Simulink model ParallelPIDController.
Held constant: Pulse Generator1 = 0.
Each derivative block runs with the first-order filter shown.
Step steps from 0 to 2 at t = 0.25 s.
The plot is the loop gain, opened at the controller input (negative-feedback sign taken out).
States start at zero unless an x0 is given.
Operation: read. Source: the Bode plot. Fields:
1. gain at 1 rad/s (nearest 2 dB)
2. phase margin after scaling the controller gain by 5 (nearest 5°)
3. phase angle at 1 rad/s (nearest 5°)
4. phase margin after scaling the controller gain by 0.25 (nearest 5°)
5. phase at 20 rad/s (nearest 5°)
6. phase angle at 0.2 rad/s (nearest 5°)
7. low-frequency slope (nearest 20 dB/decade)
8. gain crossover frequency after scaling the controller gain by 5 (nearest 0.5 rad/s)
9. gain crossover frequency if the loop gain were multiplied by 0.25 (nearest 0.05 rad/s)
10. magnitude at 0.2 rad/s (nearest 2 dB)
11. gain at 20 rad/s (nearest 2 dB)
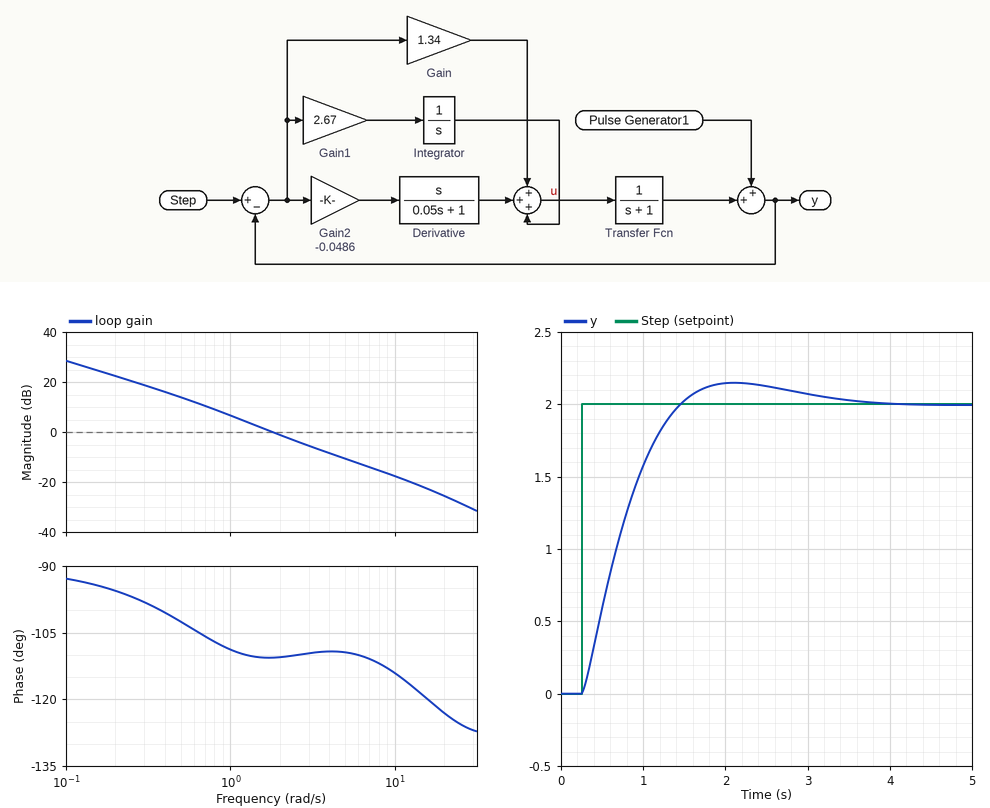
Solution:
6 dB
70°
-110°
75°
-125°
-95°
-20 dB/decade
7.0 rad/s
0.60 rad/s
22 dB
-26 dB
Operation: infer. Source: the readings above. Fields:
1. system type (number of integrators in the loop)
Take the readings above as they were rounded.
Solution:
1
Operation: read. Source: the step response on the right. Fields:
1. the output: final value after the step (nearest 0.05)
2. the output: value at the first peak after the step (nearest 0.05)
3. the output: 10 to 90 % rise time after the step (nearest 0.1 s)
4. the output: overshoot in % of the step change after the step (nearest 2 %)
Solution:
2.00
2.15
0.8 s
8 %
